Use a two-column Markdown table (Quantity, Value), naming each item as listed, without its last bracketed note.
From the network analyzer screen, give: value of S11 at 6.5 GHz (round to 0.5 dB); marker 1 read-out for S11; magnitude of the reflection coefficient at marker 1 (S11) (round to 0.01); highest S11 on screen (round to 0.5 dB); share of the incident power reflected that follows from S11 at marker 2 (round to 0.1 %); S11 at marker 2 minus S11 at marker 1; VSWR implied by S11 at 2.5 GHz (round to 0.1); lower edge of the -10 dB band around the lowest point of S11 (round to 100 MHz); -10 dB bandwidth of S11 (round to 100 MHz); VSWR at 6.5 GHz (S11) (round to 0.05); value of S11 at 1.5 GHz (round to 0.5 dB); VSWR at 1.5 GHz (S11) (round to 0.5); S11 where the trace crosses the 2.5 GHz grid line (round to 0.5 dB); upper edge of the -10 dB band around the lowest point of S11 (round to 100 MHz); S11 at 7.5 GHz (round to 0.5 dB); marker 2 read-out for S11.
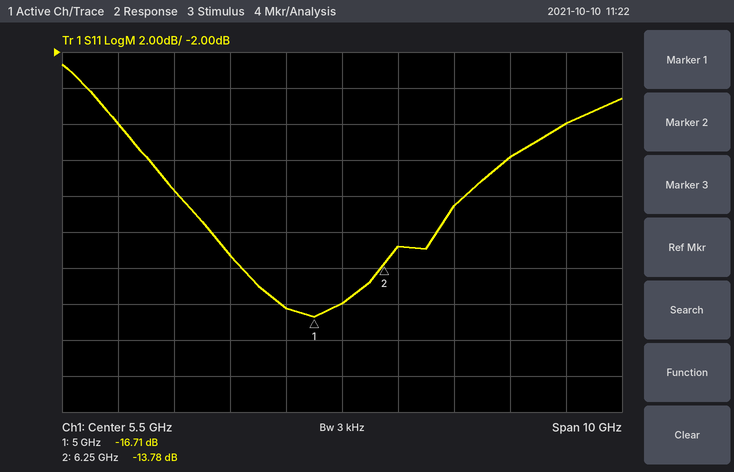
| Quantity | Value |
|---|---|
| value of S11 at 6.5 GHz | -13.0 dB |
| marker 1 read-out for S11 | -16.71 dB |
| magnitude of the reflection coefficient at marker 1 (S11) | 0.15 |
| highest S11 on screen | -2.5 dB |
| share of the incident power reflected that follows from S11 at marker 2 | 4.2 % |
| S11 at marker 2 minus S11 at marker 1 | 2.93 dB |
| VSWR implied by S11 at 2.5 GHz | 2.0 |
| lower edge of the -10 dB band around the lowest point of S11 | 2.6 GHz |
| -10 dB bandwidth of S11 | 5.1 GHz |
| VSWR at 6.5 GHz (S11) | 1.60 |
| value of S11 at 1.5 GHz | -6.0 dB |
| VSWR at 1.5 GHz (S11) | 3.0 |
| S11 where the trace crosses the 2.5 GHz grid line | -9.5 dB |
| upper edge of the -10 dB band around the lowest point of S11 | 7.7 GHz |
| S11 at 7.5 GHz | -10.5 dB |
| marker 2 read-out for S11 | -13.78 dB |
